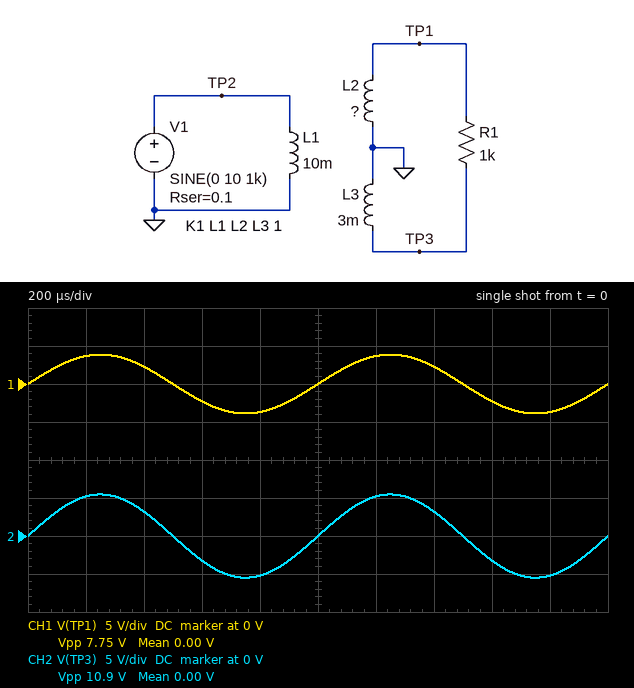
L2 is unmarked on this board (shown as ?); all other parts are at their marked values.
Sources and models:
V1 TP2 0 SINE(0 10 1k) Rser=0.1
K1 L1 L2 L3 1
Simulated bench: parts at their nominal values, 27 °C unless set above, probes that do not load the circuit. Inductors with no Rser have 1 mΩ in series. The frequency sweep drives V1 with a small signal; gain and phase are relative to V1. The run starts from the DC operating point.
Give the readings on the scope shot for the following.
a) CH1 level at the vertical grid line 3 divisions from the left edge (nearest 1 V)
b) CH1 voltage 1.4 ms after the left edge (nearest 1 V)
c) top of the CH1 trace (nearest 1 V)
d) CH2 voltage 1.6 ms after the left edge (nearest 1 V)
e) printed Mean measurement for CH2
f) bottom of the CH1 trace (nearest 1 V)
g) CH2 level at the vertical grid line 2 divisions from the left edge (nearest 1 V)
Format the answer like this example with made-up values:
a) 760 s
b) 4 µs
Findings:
a) -2 V
b) 2 V
c) 4 V
d) -3 V
e) 0.00 V
f) -4 V
g) 3 V
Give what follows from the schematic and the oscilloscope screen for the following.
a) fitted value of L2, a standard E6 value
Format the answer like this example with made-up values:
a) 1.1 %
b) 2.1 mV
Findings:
a) 1.5 mH
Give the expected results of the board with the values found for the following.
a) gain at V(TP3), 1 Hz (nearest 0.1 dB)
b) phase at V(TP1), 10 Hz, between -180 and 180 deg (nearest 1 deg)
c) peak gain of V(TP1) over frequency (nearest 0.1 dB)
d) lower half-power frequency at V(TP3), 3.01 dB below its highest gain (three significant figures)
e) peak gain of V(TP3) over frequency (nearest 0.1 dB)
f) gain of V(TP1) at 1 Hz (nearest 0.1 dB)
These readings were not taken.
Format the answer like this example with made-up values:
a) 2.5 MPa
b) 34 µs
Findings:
a) -10.8 dB
b) 9 deg
c) -8.2 dB
d) 1.61 Hz
e) -5.2 dB
f) -13.8 dB
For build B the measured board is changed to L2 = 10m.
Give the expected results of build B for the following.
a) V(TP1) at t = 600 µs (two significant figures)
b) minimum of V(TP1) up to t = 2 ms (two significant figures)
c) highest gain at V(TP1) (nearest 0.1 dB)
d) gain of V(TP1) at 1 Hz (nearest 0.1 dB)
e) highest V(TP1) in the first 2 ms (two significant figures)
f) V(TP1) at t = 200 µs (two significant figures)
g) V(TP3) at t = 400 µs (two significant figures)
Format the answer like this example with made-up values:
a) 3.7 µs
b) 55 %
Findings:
a) -5.9 V
b) -10 V
c) 0 dB
d) -5.5 dB
e) 10 V
f) 9.5 V
g) 3.2 V
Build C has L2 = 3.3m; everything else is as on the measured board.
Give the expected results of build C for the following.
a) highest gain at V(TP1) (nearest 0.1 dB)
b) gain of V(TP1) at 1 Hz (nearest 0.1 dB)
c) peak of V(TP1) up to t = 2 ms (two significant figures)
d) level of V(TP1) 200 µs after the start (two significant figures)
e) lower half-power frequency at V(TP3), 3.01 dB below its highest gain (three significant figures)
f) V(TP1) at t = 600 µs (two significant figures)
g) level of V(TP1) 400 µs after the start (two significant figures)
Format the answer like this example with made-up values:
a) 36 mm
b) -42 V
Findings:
a) -4.8 dB
b) -10.4 dB
c) 5.7 V
d) 5.5 V
e) 1.61 Hz
f) -3.4 V
g) 3.4 V
